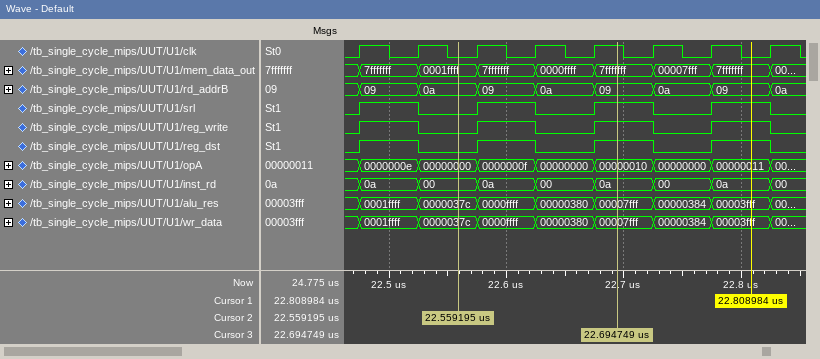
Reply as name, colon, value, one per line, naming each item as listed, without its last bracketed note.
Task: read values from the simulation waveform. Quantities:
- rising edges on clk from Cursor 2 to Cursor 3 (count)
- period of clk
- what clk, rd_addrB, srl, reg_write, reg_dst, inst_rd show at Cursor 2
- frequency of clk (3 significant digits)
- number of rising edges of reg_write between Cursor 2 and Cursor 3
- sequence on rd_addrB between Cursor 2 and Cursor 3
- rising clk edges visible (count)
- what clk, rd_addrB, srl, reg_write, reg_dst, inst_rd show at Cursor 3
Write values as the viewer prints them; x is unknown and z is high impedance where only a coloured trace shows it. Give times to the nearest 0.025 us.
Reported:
rising edges on clk from Cursor 2 to Cursor 3: 3
period of clk: 0.05 us
what clk, rd_addrB, srl, reg_write, reg_dst, inst_rd show at Cursor 2: clk=0, rd_addrB=0a, srl=0, reg_write=0, reg_dst=0, inst_rd=00
frequency of clk: 20.0 MHz
number of rising edges of reg_write between Cursor 2 and Cursor 3: 2
sequence on rd_addrB between Cursor 2 and Cursor 3: 0a, 09, 0a, 09
rising clk edges visible: 8
what clk, rd_addrB, srl, reg_write, reg_dst, inst_rd show at Cursor 3: clk=1, rd_addrB=09, srl=1, reg_write=1, reg_dst=1, inst_rd=0a
